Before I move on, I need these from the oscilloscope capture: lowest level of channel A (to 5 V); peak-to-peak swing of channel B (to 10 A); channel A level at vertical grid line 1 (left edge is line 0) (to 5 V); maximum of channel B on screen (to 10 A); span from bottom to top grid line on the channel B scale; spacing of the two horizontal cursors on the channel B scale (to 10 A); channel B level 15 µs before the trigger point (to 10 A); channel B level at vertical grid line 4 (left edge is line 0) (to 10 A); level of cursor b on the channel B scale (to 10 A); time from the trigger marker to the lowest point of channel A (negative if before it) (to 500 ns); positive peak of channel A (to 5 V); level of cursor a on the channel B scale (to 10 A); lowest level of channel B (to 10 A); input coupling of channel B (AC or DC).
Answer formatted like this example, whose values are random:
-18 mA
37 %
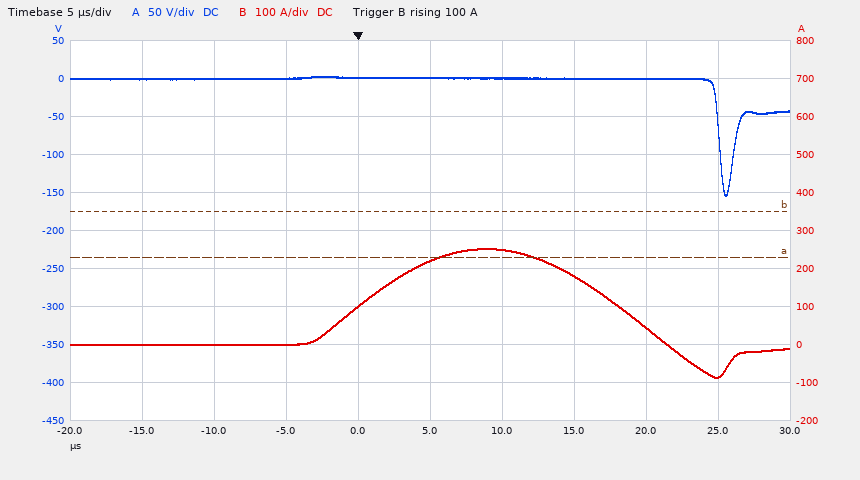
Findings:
-155 V
340 A
0 V
250 A
1 kA
120 A
0 A
100 A
350 A
+25.5 µs
5 V
230 A
-90 A
DC
